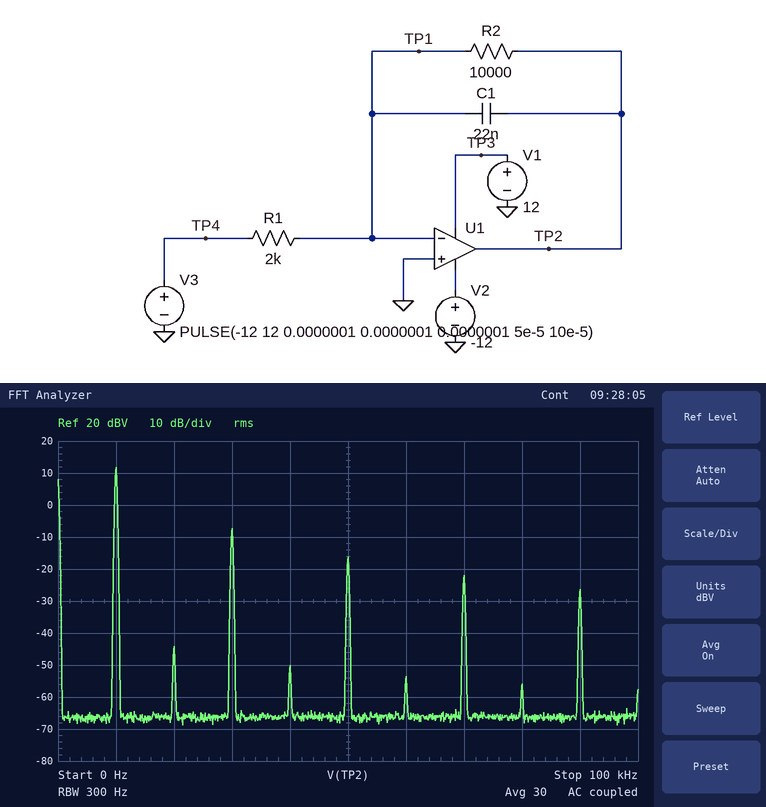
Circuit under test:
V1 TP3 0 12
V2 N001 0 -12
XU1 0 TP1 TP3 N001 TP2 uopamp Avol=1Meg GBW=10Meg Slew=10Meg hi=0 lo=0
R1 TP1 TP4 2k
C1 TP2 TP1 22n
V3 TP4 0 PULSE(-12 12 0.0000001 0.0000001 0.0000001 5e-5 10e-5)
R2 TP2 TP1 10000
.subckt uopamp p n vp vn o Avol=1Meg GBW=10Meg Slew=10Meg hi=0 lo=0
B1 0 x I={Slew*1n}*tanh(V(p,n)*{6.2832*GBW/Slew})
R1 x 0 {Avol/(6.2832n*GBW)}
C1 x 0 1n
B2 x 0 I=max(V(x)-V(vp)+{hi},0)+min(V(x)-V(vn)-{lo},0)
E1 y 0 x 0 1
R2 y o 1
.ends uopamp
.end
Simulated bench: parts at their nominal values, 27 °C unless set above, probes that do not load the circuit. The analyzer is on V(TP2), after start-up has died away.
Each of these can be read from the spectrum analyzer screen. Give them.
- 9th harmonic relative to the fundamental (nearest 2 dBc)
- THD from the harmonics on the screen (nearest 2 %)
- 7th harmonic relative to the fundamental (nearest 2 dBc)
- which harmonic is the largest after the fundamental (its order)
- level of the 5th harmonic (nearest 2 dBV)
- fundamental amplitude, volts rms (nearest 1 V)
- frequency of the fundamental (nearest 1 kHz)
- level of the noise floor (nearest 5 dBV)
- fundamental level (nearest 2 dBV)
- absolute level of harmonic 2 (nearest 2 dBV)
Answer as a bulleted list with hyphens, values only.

- -38 dBc
- 12 %
- -34 dBc
- 3
- -16 dBV
- 4 V
- 10 kHz
- -65 dBV
- 12 dBV
- -44 dBV
